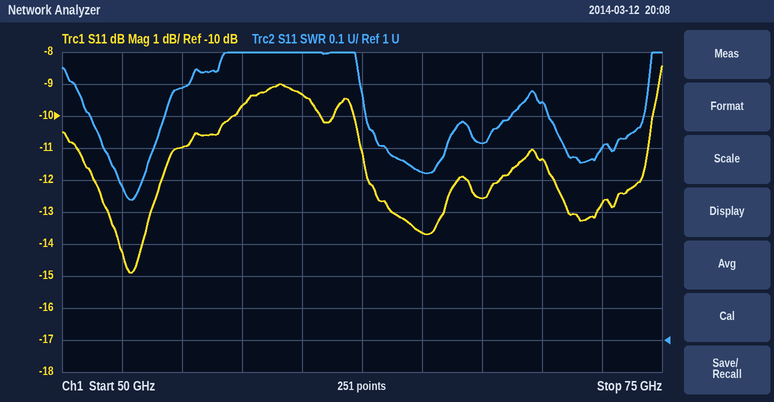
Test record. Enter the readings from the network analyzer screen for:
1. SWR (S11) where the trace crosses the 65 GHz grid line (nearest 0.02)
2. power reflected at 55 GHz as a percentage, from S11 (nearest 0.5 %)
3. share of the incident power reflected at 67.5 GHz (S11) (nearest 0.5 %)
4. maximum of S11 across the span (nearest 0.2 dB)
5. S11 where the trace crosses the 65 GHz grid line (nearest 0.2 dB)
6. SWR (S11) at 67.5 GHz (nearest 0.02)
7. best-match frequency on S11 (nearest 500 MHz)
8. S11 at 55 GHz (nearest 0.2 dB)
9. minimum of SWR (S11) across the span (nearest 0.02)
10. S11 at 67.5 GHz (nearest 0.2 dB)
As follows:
1.52
8.0 %
5.5 %
-8.4 dB
-13.6 dB
1.62
53.0 GHz
-11.0 dB
1.44
-12.6 dB
